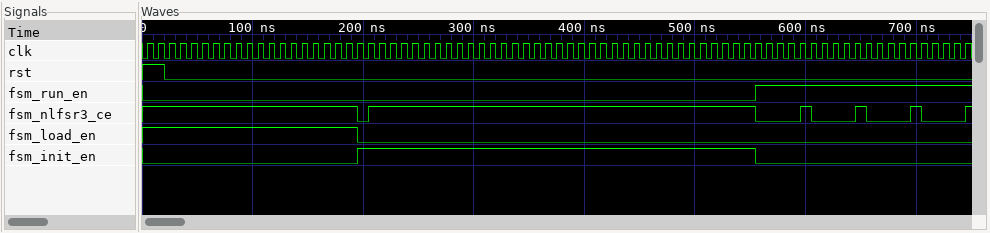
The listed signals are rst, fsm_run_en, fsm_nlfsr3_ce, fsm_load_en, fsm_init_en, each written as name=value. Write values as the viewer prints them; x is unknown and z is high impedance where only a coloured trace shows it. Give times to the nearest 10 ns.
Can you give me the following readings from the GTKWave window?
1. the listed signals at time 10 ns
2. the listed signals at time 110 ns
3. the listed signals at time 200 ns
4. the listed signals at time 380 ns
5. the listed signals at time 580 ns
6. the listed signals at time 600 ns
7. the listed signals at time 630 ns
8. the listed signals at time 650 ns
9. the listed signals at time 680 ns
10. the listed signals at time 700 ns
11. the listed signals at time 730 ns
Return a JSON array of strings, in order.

["rst=1, fsm_run_en=0, fsm_nlfsr3_ce=1, fsm_load_en=1, fsm_init_en=0", "rst=0, fsm_run_en=0, fsm_nlfsr3_ce=1, fsm_load_en=1, fsm_init_en=0", "rst=0, fsm_run_en=0, fsm_nlfsr3_ce=0, fsm_load_en=0, fsm_init_en=1", "rst=0, fsm_run_en=0, fsm_nlfsr3_ce=1, fsm_load_en=0, fsm_init_en=1", "rst=0, fsm_run_en=1, fsm_nlfsr3_ce=0, fsm_load_en=0, fsm_init_en=0", "rst=0, fsm_run_en=1, fsm_nlfsr3_ce=1, fsm_load_en=0, fsm_init_en=0", "rst=0, fsm_run_en=1, fsm_nlfsr3_ce=0, fsm_load_en=0, fsm_init_en=0", "rst=0, fsm_run_en=1, fsm_nlfsr3_ce=1, fsm_load_en=0, fsm_init_en=0", "rst=0, fsm_run_en=1, fsm_nlfsr3_ce=0, fsm_load_en=0, fsm_init_en=0", "rst=0, fsm_run_en=1, fsm_nlfsr3_ce=1, fsm_load_en=0, fsm_init_en=0", "rst=0, fsm_run_en=1, fsm_nlfsr3_ce=0, fsm_load_en=0, fsm_init_en=0"]
